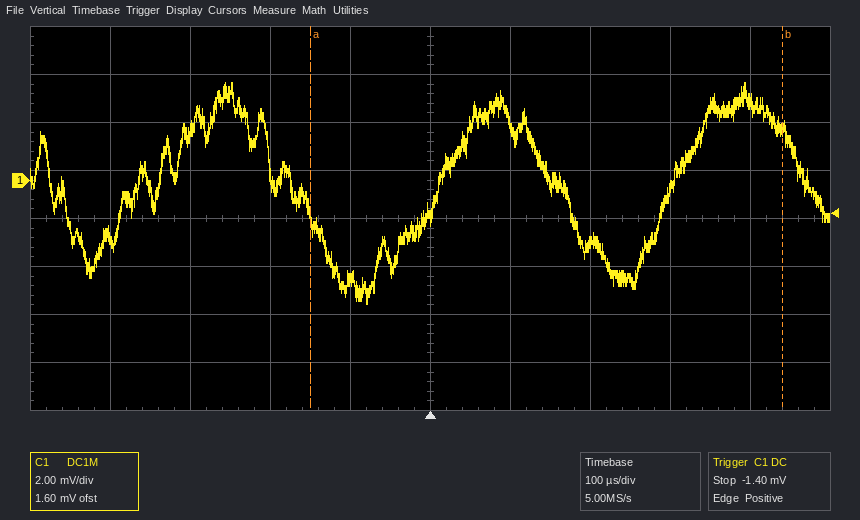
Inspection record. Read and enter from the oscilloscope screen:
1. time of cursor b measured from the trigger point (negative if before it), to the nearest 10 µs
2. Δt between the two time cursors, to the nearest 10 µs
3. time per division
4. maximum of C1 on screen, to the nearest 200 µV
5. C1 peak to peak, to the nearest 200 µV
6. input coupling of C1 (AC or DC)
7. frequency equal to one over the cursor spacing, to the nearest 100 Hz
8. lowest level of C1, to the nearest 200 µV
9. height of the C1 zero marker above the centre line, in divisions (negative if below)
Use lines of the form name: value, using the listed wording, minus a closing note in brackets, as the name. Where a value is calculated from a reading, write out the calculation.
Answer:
time of cursor b measured from the trigger point (negative if before it), to the nearest 10 µs: +440 µs
Δt between the two time cursors, to the nearest 10 µs: 590 µs
time per division: 100 µs
maximum of C1 on screen, to the nearest 200 µV: 4.0 mV
C1 peak to peak, to the nearest 200 µV: 4.0 mV − (-5.2 mV) = 9.2 mV
input coupling of C1: DC
frequency equal to one over the cursor spacing, to the nearest 100 Hz: 1 / 590 µs ≈ 1.7 kHz
lowest level of C1, to the nearest 200 µV: -5.2 mV
height of the C1 zero marker above the centre line, in divisions: +0.8 div
